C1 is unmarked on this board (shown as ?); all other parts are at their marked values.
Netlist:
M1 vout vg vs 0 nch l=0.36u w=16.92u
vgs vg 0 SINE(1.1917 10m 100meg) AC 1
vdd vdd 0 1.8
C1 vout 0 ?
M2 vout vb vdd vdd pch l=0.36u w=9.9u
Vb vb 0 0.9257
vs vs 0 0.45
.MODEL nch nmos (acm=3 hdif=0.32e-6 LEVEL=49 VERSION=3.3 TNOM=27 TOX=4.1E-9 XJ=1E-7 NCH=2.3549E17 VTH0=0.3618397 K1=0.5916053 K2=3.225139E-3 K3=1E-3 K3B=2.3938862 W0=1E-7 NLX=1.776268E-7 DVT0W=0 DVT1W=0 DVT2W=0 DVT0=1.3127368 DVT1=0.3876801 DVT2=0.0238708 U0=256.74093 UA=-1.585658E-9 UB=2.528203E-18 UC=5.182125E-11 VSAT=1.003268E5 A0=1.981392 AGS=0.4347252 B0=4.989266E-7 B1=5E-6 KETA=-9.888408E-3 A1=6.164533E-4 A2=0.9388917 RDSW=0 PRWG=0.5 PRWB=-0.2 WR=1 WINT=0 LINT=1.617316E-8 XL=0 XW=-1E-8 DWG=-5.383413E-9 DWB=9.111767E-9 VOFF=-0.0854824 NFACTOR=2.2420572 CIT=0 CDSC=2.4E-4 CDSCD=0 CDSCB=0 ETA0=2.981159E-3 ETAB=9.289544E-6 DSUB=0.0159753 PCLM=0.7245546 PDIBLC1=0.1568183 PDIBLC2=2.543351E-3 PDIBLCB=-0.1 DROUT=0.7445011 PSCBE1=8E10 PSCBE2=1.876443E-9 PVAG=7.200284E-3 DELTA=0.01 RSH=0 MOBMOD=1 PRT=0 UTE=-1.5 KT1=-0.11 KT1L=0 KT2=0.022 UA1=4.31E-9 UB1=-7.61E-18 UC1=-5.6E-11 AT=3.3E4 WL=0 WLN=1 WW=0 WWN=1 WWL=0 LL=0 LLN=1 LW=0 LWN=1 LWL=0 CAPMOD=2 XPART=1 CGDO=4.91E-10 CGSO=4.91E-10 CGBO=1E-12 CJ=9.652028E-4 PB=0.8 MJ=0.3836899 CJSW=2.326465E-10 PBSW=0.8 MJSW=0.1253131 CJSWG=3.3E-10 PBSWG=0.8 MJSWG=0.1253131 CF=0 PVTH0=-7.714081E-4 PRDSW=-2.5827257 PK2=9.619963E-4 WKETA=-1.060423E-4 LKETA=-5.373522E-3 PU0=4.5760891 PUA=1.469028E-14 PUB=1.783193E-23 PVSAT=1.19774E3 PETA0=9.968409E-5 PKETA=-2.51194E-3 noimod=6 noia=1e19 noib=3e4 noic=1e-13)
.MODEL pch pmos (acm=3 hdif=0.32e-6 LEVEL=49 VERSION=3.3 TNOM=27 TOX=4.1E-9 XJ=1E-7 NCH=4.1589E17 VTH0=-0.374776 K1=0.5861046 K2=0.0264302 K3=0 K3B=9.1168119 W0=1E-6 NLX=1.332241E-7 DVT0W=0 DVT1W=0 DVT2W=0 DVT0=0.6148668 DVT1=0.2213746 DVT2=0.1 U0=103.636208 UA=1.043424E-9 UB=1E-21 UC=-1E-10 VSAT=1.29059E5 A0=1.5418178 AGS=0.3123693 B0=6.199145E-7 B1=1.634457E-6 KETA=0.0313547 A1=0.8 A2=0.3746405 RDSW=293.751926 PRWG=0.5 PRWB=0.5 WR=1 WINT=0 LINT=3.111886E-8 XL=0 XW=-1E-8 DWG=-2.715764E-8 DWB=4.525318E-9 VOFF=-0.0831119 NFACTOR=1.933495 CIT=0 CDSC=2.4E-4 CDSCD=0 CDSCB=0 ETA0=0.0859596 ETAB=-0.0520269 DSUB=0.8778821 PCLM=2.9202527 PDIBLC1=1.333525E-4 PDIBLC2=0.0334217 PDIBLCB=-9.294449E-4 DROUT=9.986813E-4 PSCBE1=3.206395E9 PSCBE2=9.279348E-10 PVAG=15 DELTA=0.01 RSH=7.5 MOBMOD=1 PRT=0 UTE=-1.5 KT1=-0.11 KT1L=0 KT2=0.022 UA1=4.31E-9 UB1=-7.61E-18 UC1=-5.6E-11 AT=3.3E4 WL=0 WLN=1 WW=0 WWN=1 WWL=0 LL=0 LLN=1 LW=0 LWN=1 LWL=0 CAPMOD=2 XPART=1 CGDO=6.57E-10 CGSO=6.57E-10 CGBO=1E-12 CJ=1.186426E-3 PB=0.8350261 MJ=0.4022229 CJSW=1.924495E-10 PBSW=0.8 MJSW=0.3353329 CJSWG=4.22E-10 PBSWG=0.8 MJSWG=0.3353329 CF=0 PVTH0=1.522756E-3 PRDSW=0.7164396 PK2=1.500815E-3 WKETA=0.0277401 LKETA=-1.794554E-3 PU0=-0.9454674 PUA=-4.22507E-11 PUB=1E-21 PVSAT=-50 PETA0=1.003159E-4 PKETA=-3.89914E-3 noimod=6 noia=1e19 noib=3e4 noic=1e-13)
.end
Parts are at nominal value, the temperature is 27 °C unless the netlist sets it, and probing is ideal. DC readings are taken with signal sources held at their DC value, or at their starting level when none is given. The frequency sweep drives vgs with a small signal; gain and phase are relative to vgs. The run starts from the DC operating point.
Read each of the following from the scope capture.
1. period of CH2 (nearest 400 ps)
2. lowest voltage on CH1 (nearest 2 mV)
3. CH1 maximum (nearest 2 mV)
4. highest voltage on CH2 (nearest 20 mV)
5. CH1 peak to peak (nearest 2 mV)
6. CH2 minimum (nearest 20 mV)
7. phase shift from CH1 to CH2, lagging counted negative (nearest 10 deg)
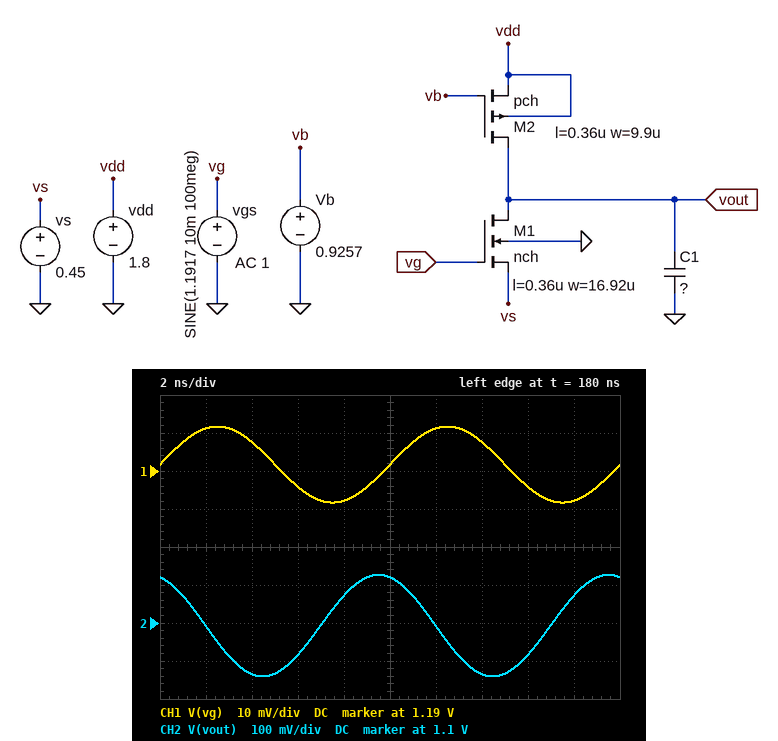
10.0 ns
1.182 V
1.202 V
1.22 V
20 mV
960 mV
110 deg
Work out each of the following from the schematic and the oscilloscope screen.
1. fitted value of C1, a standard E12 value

180 fF
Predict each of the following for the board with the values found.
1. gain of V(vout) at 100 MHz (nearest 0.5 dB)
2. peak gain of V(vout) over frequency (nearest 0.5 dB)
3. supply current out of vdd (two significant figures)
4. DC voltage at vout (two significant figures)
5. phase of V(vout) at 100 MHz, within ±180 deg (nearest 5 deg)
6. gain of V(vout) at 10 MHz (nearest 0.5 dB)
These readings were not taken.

22.5 dB
32.5 dB
170 µA
1.1 V
110 deg
32.0 dB
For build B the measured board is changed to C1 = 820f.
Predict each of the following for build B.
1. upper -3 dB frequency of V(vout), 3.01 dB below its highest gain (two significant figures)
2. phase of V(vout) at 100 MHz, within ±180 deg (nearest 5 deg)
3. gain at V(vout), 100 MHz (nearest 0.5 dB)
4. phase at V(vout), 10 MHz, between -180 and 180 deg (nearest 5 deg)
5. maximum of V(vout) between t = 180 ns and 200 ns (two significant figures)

8.7 MHz
95 deg
11.0 dB
130 deg
1.1 V
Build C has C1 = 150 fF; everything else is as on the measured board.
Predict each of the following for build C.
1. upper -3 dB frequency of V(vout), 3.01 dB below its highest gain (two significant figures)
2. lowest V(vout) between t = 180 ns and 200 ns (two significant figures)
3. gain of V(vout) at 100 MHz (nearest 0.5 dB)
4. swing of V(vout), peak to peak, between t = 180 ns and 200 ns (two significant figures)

39 MHz
940 mV
23.5 dB
300 mV
